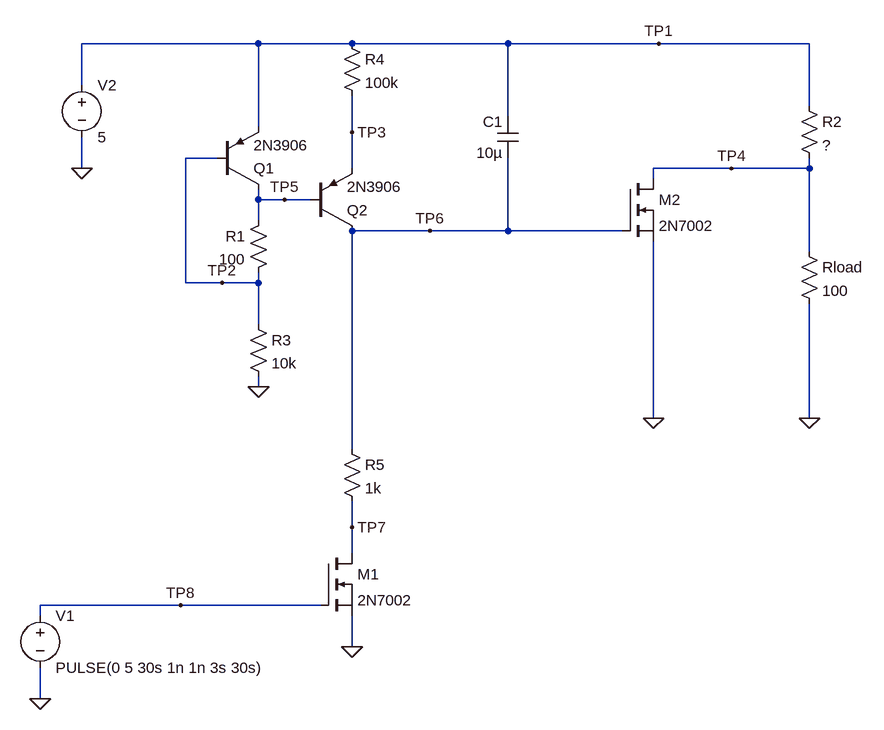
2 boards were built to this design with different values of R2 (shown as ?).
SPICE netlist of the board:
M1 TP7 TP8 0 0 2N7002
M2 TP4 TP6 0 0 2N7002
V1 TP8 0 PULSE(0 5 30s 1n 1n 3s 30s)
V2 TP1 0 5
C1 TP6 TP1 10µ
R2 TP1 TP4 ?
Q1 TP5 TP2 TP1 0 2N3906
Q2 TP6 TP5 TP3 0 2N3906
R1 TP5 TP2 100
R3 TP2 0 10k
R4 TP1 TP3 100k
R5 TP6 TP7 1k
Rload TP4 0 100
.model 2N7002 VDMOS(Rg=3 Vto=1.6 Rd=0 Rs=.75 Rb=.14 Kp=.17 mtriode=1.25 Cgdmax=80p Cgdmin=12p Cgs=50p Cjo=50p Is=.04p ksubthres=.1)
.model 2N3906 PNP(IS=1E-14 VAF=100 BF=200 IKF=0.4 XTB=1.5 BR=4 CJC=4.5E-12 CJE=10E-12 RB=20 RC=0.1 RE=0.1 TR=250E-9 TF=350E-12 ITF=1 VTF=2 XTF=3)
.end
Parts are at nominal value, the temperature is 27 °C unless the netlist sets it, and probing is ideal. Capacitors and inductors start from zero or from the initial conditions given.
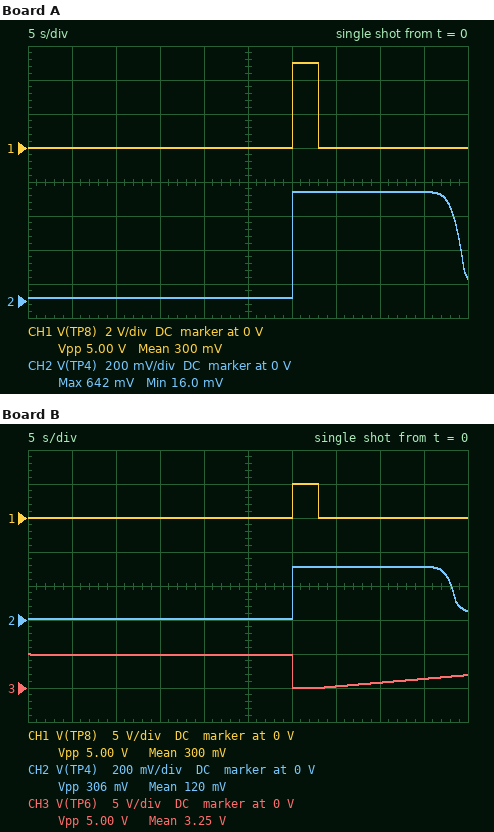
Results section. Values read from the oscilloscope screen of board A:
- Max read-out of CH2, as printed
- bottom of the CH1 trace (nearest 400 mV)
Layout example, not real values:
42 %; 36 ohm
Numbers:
642 mV; 0 V
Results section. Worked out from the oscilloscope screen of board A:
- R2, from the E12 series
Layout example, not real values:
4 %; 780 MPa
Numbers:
680 Ω
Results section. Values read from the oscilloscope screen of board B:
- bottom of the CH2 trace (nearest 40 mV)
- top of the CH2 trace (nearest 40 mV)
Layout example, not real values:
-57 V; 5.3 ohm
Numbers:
0 V; 320 mV
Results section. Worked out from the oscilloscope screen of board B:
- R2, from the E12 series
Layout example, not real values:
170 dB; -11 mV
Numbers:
1.5 kΩ
